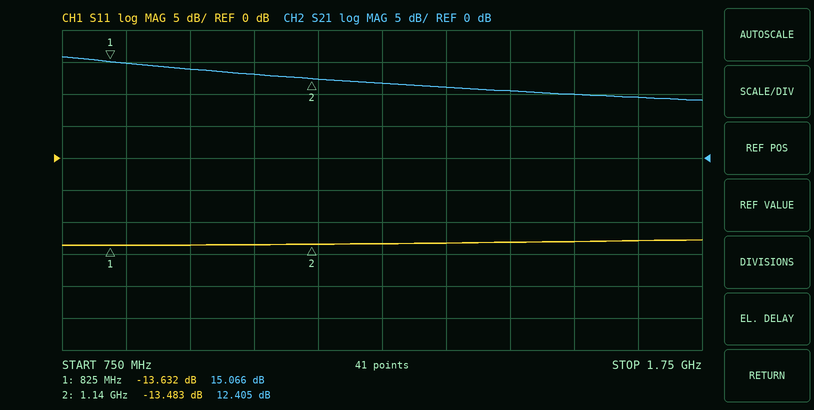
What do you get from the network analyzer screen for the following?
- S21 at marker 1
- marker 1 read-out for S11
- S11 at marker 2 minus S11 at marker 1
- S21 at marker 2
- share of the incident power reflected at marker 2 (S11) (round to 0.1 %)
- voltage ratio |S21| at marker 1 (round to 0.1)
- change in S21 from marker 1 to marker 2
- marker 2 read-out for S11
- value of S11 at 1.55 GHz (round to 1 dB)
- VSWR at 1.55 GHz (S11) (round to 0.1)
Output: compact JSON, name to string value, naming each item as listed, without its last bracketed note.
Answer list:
{"S21 at marker 1": "15.066 dB", "marker 1 read-out for S11": "-13.632 dB", "S11 at marker 2 minus S11 at marker 1": "0.149 dB", "S21 at marker 2": "12.405 dB", "share of the incident power reflected at marker 2 (S11)": "4.5 %", "voltage ratio |S21| at marker 1": "5.7", "change in S21 from marker 1 to marker 2": "-2.661 dB", "marker 2 read-out for S11": "-13.483 dB", "value of S11 at 1.55 GHz": "-13 dB", "VSWR at 1.55 GHz (S11)": "1.6"}
